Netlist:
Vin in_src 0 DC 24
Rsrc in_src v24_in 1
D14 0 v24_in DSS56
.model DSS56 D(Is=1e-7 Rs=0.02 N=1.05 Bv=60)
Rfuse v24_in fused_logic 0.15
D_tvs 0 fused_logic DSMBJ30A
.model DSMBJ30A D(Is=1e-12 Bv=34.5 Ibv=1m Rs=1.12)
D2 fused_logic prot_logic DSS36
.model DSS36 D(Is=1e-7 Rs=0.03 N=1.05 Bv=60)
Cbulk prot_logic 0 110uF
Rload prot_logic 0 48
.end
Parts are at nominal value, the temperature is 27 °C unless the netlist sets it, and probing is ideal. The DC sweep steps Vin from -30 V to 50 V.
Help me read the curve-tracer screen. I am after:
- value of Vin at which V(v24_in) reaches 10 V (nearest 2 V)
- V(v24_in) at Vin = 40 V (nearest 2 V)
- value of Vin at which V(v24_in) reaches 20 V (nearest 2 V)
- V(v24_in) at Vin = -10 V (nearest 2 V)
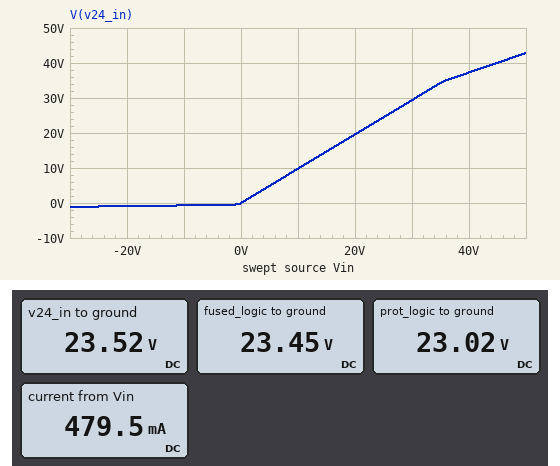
10 V
38 V
20 V
0 V
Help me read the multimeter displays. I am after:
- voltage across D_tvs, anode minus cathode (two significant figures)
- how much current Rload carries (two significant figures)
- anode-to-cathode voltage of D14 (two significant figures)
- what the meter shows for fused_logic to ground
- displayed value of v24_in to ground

-23 V
480 mA
-24 V
23.45 V
23.52 V
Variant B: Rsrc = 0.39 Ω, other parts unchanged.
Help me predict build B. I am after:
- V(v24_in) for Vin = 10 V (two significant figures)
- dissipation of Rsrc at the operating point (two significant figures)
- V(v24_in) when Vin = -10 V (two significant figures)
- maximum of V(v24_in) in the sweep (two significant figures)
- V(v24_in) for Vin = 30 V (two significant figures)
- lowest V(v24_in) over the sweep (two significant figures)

9.9 V
92 mW
-980 mV
46 V
30 V
-2.0 V
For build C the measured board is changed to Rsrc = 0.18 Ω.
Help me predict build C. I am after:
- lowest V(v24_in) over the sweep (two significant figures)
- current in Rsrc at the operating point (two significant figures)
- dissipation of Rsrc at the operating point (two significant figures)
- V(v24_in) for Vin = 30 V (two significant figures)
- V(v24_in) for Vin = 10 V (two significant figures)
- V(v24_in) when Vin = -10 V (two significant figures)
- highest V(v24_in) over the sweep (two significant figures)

-3.5 V
490 mA
43 mW
30 V
10 V
-1.5 V
48 V
